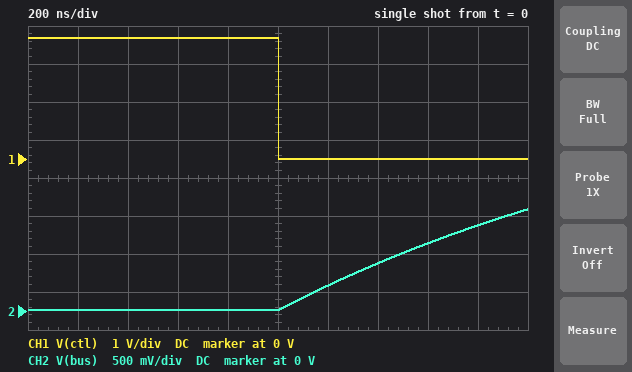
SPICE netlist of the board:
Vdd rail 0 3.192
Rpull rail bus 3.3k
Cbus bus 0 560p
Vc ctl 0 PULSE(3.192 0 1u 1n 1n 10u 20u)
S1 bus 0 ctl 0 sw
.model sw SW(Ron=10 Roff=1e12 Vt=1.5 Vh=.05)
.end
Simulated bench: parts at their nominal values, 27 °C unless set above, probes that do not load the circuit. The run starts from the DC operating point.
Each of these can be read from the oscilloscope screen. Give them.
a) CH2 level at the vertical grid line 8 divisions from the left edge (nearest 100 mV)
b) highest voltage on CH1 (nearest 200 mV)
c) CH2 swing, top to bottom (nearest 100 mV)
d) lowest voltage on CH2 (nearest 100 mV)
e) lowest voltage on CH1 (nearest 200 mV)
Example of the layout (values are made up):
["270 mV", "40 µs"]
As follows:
["900 mV", "3.2 V", "1.3 V", "0 V", "0 V"]
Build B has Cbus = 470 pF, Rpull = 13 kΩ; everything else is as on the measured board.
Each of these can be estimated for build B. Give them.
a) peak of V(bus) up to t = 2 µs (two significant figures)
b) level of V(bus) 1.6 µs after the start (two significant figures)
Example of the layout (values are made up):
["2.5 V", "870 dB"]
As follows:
["480 mV", "300 mV"]
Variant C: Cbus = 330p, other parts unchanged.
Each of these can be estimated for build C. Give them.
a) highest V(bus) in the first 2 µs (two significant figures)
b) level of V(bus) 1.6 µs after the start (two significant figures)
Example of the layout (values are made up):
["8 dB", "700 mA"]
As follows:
["1.9 V", "1.4 V"]
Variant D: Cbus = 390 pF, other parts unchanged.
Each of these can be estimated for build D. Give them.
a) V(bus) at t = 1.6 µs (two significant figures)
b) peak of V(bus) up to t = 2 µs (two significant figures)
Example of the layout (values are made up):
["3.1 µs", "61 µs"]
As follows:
["1.2 V", "1.7 V"]
